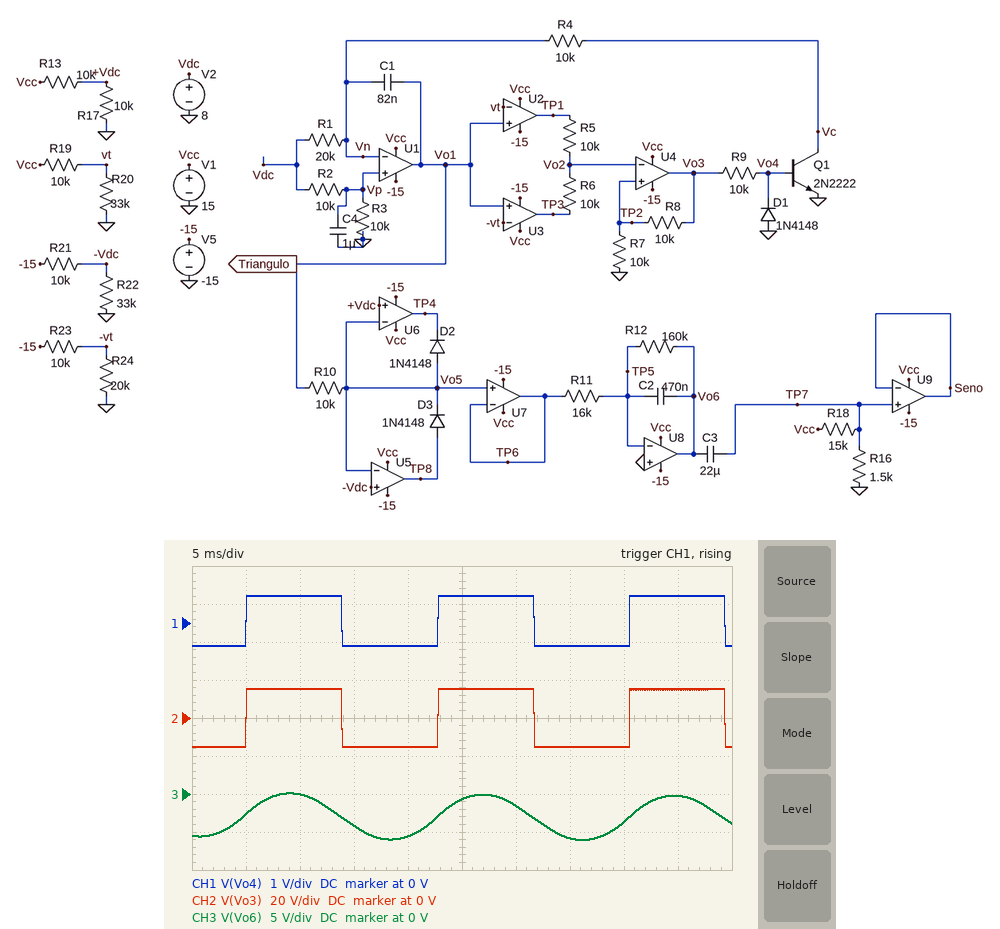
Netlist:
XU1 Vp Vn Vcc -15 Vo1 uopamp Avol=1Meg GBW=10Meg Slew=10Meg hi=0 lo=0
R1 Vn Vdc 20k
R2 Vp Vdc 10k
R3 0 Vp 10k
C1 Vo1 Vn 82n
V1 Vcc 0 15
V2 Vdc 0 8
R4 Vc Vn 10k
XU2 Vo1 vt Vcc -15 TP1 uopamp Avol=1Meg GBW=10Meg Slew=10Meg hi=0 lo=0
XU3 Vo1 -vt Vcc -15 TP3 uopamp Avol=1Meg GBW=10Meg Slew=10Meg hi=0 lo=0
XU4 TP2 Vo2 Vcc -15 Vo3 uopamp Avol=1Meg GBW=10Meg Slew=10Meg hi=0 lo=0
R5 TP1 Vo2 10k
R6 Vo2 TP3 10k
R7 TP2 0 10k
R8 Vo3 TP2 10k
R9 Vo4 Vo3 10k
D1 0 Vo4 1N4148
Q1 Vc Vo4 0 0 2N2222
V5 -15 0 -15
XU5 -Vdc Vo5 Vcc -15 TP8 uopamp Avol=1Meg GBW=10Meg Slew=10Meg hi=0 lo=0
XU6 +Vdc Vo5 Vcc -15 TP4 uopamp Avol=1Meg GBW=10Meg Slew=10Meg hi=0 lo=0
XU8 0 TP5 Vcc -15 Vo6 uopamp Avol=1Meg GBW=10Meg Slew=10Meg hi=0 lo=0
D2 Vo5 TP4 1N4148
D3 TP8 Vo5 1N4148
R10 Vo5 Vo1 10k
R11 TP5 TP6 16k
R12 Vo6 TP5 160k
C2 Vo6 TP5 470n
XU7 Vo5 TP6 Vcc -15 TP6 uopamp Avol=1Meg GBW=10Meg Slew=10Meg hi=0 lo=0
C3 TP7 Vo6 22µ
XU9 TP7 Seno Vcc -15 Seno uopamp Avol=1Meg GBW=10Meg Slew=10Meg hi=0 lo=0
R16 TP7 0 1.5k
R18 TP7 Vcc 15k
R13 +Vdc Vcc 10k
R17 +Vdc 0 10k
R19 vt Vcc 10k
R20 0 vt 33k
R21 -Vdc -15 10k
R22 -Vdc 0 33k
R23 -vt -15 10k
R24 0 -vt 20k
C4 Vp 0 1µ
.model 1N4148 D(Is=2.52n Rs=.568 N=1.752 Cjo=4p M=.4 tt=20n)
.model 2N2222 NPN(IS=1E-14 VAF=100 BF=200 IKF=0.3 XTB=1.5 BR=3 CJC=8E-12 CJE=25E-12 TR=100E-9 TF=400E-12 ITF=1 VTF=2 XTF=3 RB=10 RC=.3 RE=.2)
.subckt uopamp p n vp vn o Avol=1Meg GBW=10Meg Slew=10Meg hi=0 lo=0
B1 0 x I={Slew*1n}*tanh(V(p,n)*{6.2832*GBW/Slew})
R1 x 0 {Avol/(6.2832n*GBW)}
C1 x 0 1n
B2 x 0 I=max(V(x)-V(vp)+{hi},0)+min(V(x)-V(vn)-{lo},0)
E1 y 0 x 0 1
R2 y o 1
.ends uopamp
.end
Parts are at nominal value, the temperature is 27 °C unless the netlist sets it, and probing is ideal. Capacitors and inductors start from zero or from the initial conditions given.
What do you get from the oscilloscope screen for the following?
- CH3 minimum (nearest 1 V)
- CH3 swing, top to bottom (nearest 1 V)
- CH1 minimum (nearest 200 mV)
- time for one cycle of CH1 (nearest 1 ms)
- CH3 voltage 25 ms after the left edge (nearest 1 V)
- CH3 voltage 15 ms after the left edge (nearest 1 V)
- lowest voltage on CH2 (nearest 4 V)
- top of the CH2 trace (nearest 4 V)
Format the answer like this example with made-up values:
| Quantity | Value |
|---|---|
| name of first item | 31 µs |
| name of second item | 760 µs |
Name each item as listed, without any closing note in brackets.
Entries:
| Quantity | Value |
|---|---|
| CH3 minimum | -6 V |
| CH3 swing, top to bottom | 6 V |
| CH1 minimum | -600 mV |
| time for one cycle of CH1 | 18 ms |
| CH3 voltage 25 ms after the left edge | -1 V |
| CH3 voltage 15 ms after the left edge | -4 V |
| lowest voltage on CH2 | -16 V |
| top of the CH2 trace | 16 V |
